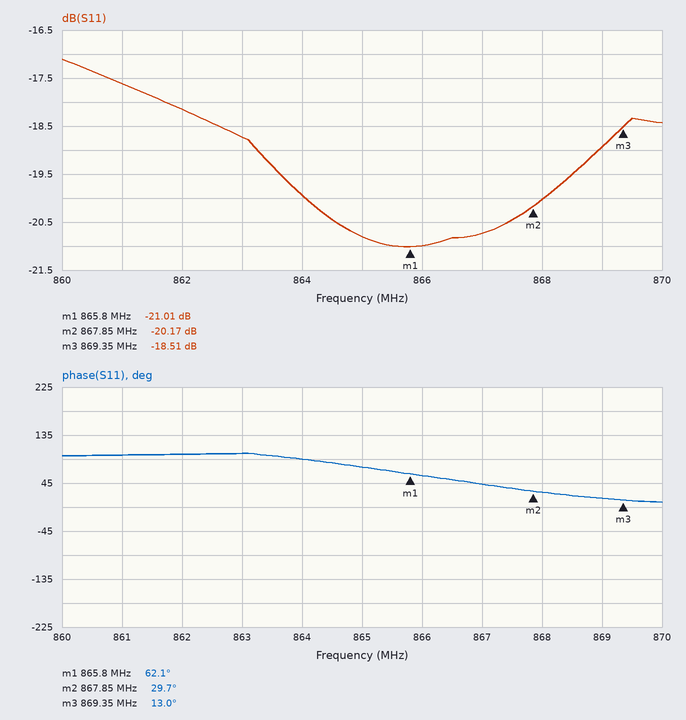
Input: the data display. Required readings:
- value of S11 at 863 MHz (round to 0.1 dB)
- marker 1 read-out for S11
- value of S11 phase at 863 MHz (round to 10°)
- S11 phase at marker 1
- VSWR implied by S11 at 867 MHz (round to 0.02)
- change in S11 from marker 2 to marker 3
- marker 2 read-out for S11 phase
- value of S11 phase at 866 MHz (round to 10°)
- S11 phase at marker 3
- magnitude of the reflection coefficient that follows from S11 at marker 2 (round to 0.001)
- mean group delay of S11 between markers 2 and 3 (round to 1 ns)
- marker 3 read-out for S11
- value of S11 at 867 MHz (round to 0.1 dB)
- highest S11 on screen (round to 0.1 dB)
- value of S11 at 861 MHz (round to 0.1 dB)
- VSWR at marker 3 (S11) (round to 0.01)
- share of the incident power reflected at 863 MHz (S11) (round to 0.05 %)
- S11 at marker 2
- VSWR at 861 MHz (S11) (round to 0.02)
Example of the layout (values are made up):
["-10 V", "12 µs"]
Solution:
["-18.7 dB", "-21.01 dB", "100°", "62.1°", "1.20", "1.66 dB", "29.7°", "60°", "13.0°", "0.098", "31 ns", "-18.51 dB", "-20.7 dB", "-17.1 dB", "-17.6 dB", "1.27", "1.35 %", "-20.17 dB", "1.30"]
